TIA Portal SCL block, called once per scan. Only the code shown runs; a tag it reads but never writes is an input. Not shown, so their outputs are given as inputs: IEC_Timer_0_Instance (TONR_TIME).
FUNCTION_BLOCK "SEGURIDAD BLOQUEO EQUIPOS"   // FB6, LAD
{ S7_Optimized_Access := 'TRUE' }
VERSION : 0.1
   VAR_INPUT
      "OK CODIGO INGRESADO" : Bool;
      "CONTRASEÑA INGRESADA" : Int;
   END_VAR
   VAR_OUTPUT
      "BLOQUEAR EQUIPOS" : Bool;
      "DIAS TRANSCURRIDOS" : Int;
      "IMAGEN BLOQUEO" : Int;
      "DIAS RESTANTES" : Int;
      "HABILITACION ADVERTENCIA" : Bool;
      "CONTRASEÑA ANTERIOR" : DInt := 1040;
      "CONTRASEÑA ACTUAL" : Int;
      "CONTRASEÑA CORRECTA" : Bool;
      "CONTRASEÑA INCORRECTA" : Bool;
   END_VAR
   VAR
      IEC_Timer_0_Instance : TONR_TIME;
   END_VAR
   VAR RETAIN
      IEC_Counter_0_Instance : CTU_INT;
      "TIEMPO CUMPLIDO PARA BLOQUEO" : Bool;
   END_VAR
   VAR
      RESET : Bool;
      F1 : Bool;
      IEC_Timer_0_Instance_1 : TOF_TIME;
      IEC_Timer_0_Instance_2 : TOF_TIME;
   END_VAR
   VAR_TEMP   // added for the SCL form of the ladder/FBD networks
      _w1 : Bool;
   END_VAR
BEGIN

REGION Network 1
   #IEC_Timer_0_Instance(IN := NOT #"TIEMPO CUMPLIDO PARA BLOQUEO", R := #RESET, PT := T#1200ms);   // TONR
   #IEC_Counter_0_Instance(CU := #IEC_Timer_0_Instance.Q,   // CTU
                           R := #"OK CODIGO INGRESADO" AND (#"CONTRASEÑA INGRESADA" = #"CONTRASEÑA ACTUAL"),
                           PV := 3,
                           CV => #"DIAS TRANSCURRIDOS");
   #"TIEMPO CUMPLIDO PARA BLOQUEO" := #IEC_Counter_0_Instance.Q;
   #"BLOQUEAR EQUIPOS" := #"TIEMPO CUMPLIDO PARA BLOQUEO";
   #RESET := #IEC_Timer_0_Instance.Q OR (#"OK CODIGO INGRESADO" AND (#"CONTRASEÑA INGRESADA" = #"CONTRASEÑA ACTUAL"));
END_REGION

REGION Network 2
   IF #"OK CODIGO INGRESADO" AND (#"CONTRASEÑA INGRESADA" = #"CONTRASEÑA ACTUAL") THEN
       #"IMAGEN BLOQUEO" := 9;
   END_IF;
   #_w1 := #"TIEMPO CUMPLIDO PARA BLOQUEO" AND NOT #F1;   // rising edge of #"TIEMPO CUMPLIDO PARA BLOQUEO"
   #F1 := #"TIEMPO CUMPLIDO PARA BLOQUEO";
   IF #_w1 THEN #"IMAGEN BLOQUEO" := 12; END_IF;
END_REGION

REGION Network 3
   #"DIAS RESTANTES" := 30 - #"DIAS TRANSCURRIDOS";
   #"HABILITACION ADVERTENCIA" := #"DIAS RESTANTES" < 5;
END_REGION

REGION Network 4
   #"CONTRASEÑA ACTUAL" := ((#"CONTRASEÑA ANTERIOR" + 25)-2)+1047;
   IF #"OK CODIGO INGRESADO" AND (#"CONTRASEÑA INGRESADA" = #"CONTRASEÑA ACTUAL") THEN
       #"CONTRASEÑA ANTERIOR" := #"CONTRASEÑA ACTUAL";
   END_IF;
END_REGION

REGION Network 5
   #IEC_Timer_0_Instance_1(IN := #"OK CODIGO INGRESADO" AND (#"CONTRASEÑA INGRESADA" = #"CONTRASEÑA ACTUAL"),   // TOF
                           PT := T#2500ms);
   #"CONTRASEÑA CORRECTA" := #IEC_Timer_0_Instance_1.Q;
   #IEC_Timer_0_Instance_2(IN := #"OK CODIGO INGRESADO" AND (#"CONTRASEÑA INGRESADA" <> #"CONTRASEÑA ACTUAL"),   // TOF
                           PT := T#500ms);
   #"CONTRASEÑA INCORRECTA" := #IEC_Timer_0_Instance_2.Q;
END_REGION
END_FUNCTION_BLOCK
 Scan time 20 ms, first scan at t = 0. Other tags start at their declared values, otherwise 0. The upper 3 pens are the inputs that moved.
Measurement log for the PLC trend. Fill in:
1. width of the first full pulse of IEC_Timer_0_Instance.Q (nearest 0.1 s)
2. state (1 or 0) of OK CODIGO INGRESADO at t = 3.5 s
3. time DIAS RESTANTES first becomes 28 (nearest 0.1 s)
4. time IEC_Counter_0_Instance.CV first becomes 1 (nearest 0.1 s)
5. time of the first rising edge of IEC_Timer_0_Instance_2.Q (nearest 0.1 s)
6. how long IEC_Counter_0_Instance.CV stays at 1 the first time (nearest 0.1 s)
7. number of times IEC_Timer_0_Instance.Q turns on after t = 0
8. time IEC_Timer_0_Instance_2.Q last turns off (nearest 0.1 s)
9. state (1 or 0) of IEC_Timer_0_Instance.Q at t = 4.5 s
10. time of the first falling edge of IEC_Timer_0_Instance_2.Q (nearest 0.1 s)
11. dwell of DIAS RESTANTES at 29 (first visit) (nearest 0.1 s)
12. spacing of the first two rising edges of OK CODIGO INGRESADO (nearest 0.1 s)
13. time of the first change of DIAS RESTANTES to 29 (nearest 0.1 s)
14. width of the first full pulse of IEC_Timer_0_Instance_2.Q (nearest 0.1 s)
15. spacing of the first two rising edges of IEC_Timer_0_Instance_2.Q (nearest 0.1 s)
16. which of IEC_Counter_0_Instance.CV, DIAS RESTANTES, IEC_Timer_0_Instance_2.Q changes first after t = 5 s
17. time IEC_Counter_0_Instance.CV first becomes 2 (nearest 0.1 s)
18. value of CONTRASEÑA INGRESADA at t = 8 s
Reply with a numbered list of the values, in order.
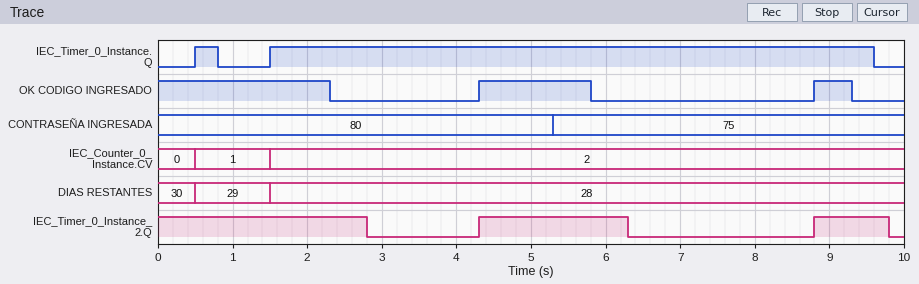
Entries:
1. 0.3 s
2. 0
3. 1.5 s
4. 0.5 s
5. 4.3 s
6. 1.0 s
7. 2
8. 9.8 s
9. 1
10. 2.8 s
11. 1.0 s
12. 4.5 s
13. 0.5 s
14. 2.0 s
15. 4.5 s
16. IEC_Timer_0_Instance_2.Q
17. 1.5 s
18. 75
